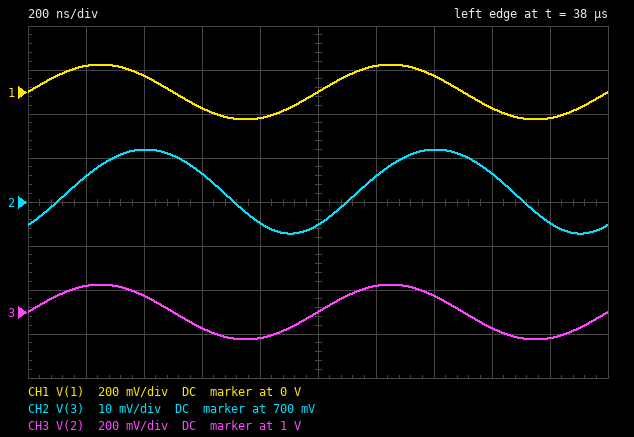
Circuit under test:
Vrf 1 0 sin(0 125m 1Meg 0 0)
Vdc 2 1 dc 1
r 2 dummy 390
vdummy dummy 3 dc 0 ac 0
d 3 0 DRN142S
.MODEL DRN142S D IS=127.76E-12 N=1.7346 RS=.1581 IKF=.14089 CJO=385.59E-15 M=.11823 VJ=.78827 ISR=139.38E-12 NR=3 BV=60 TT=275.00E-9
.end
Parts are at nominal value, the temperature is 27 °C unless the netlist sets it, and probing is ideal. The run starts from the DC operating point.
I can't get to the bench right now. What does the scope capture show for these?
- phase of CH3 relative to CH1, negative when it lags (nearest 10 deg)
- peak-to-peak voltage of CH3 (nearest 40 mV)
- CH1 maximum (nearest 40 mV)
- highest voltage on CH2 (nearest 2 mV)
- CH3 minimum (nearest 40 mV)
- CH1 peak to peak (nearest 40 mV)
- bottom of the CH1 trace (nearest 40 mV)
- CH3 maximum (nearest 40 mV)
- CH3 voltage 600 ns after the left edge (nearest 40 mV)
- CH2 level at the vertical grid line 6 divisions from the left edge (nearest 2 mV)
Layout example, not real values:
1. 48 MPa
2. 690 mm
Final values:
1. 0 deg
2. 240 mV
3. 120 mV
4. 712 mV
5. 880 mV
6. 240 mV
7. -120 mV
8. 1.12 V
9. 920 mV
10. 706 mV
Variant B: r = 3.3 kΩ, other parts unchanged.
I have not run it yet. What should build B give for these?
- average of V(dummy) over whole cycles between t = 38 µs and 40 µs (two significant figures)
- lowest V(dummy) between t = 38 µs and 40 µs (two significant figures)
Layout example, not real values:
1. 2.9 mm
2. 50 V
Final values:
1. 620 mV
2. 610 mV
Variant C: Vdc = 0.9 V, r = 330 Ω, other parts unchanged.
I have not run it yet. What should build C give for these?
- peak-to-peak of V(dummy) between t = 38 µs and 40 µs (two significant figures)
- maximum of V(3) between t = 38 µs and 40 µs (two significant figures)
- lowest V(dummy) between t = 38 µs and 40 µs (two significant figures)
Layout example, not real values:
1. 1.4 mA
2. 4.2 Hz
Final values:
1. 27 mV
2. 710 mV
3. 680 mV
